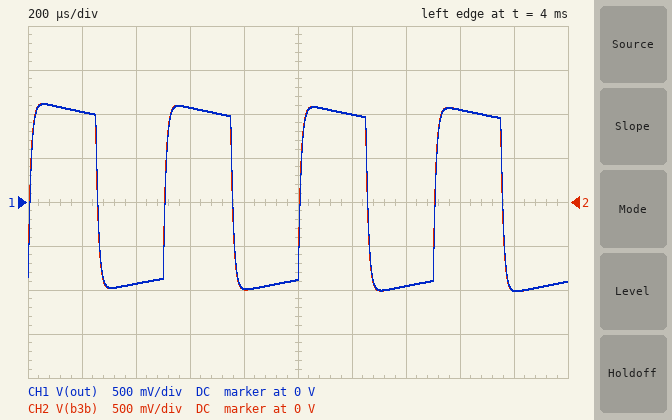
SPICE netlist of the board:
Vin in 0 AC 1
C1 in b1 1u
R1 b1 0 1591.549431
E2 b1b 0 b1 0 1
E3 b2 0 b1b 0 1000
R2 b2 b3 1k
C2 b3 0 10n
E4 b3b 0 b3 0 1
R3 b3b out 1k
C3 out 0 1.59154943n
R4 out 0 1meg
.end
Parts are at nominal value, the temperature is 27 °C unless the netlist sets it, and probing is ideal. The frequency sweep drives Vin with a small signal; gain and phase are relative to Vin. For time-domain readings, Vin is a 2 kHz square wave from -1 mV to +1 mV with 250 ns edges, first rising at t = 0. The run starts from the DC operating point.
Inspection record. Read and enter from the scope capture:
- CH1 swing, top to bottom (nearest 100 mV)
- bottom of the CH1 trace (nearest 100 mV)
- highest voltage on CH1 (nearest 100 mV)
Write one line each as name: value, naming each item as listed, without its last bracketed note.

CH1 swing, top to bottom: 2.1 V
bottom of the CH1 trace: -1.0 V
highest voltage on CH1: 1.1 V
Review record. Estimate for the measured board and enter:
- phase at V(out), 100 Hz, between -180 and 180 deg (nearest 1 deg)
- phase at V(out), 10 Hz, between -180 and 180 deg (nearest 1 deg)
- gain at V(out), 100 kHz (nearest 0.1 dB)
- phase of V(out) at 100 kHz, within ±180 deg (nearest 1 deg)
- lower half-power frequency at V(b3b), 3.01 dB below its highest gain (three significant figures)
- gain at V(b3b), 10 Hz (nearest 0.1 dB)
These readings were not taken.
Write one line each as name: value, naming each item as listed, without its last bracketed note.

phase at V(out), 100 Hz, between -180 and 180 deg: 45 deg
phase at V(out), 10 Hz, between -180 and 180 deg: 84 deg
gain at V(out), 100 kHz: 40.9 dB
phase of V(out) at 100 kHz, within ±180 deg: -126 deg
lower half-power frequency at V(b3b), 3.01 dB below its highest gain: 98.8 Hz
gain at V(b3b), 10 Hz: 40.0 dB
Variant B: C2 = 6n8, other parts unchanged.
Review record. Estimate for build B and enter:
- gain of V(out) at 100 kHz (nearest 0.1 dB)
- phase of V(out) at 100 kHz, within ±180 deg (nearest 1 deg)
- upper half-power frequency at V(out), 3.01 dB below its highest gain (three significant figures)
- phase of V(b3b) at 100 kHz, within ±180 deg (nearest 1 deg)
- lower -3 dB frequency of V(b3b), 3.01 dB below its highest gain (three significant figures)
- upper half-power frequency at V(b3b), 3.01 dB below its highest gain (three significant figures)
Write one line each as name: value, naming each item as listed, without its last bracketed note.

gain of V(out) at 100 kHz: 44.1 dB
phase of V(out) at 100 kHz, within ±180 deg: -122 deg
upper half-power frequency at V(out), 3.01 dB below its highest gain: 22.5 kHz
phase of V(b3b) at 100 kHz, within ±180 deg: -77 deg
lower -3 dB frequency of V(b3b), 3.01 dB below its highest gain: 99.2 Hz
upper half-power frequency at V(b3b), 3.01 dB below its highest gain: 23.6 kHz
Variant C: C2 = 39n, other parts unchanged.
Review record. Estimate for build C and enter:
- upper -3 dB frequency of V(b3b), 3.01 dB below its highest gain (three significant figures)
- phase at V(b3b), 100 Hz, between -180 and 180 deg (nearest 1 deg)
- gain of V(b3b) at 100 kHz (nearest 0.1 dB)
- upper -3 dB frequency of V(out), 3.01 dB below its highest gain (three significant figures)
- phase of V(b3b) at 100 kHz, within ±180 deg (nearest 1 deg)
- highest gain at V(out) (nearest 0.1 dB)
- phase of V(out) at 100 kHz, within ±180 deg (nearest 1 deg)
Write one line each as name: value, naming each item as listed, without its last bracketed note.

upper -3 dB frequency of V(b3b), 3.01 dB below its highest gain: 4.28 kHz
phase at V(b3b), 100 Hz, between -180 and 180 deg: 44 deg
gain of V(b3b) at 100 kHz: 32.2 dB
upper -3 dB frequency of V(out), 3.01 dB below its highest gain: 4.27 kHz
phase of V(b3b) at 100 kHz, within ±180 deg: -88 deg
highest gain at V(out): 59.8 dB
phase of V(out) at 100 kHz, within ±180 deg: -133 deg
